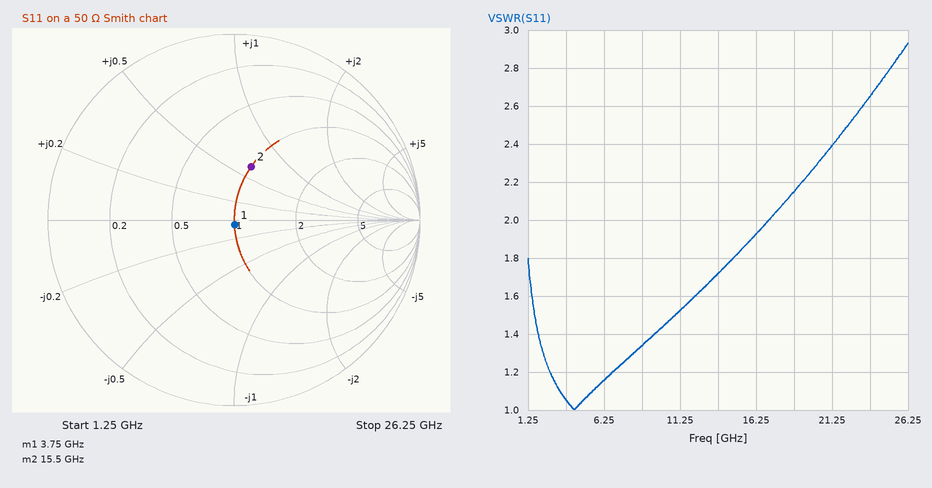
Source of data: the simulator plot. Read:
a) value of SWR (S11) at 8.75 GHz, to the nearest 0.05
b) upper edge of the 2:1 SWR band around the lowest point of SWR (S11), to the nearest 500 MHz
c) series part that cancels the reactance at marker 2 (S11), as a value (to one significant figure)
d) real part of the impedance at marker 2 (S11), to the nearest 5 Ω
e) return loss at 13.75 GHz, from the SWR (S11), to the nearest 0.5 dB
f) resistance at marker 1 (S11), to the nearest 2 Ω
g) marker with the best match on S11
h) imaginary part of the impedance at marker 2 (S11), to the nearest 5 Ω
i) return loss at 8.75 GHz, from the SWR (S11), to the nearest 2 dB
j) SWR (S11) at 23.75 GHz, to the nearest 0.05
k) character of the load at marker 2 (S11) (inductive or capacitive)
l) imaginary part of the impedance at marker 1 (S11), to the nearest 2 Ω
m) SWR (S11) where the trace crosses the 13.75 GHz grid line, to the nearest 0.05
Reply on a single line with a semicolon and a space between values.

1.35; 17.0 GHz; 300 fF; 50 Ω; 11.5 dB; 50 Ω; marker 1; +30 Ω; 16 dB; 2.65; inductive; -2 Ω; 1.70
